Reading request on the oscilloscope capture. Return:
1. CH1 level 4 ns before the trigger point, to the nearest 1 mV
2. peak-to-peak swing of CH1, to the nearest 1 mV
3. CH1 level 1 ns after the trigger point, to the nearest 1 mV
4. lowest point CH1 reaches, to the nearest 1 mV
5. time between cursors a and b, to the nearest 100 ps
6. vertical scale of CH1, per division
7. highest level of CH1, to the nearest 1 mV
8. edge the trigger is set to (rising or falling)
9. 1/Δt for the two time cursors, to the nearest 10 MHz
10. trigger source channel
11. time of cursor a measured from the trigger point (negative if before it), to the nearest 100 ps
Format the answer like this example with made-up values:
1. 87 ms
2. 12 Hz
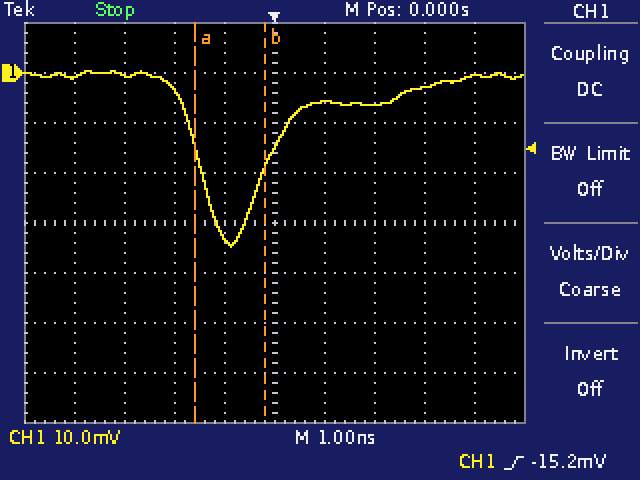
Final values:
1. -1 mV
2. 35 mV
3. -6 mV
4. -35 mV
5. 1.4 ns
6. 10 mV
7. 0 mV
8. rising
9. 710 MHz
10. CH1
11. -1.6 ns
